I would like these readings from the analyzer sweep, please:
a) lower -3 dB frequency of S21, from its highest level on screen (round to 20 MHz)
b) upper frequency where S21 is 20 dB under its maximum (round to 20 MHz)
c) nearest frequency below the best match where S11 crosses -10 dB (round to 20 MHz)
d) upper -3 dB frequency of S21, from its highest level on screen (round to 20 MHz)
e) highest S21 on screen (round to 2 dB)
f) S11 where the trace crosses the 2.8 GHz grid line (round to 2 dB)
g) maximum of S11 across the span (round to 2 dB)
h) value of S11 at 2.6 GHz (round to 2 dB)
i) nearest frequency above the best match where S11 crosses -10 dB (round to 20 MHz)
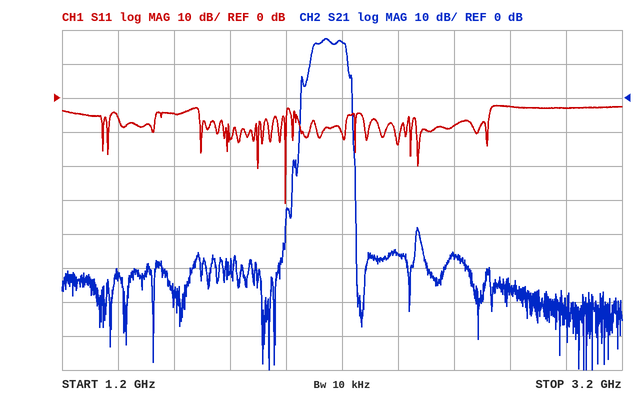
2.10 GHz
2.24 GHz
2.00 GHz
2.22 GHz
18 dB
-2 dB
-2 dB
-8 dB
2.00 GHz
